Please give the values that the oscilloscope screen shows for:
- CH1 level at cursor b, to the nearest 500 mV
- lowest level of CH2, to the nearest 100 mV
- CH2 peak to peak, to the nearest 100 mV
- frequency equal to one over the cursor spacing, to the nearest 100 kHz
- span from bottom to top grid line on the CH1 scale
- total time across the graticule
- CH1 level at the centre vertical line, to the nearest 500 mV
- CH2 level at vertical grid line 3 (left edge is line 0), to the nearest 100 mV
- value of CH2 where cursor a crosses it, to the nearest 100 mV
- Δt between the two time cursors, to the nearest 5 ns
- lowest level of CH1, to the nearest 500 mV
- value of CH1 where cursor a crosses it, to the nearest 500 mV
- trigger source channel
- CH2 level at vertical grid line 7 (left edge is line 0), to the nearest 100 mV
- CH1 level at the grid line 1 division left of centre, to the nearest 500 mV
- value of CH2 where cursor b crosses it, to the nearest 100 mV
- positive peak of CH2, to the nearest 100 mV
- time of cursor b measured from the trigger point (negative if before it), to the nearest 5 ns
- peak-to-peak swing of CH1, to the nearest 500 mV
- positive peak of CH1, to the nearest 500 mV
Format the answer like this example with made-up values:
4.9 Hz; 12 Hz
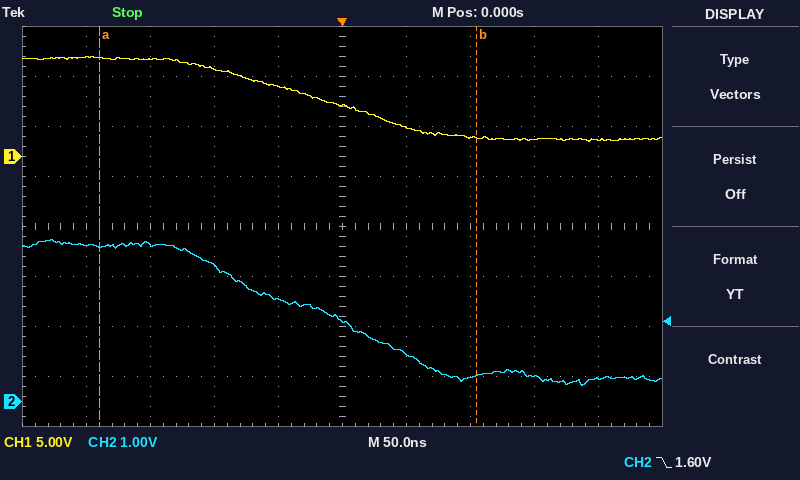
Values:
2.0 V; 300 mV; 2.9 V; 3.4 MHz; 40 V; 500 ns; 5.0 V; 2.7 V; 3.1 V; 295 ns; 1.5 V; 10.0 V; CH2; 500 mV; 7.0 V; 500 mV; 3.2 V; +105 ns; 8.5 V; 10.0 V
